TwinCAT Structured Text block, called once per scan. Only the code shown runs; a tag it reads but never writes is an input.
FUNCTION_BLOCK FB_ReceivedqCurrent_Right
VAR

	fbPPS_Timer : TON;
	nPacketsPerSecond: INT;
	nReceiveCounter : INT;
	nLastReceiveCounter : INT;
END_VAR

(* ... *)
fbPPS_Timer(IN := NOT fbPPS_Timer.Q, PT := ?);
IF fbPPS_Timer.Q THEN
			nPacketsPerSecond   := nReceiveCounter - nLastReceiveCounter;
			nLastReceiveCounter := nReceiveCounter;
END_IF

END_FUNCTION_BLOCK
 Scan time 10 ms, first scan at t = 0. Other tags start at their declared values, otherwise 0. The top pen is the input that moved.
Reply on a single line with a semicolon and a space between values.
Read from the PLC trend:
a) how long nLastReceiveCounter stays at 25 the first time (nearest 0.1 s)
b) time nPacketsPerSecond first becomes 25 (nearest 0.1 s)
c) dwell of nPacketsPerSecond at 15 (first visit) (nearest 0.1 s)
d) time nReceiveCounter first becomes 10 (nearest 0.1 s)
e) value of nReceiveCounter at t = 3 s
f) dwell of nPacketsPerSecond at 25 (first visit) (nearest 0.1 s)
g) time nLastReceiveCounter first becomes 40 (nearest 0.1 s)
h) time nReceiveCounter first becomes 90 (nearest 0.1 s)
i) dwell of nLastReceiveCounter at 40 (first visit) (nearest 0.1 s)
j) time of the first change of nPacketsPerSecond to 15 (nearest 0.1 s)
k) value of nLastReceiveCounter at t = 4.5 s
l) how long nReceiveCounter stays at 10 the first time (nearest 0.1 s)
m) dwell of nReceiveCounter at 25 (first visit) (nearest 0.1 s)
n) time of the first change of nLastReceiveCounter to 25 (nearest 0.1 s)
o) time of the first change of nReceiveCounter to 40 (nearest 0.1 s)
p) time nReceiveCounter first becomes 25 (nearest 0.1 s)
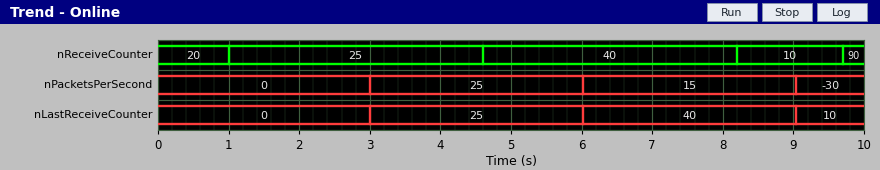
3.0 s; 3.0 s; 3.0 s; 8.2 s; 25; 3.0 s; 6.0 s; 9.7 s; 3.0 s; 6.0 s; 25; 1.5 s; 3.6 s; 3.0 s; 4.6 s; 1.0 s
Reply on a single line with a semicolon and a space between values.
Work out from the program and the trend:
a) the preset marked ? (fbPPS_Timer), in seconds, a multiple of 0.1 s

3.0 s
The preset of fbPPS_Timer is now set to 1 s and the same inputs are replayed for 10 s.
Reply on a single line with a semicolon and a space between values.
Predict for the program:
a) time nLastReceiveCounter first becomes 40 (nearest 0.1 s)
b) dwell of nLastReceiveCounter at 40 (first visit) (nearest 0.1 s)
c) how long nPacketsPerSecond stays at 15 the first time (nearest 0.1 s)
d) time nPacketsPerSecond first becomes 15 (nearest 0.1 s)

5.1 s; 4.1 s; 1.0 s; 5.1 s
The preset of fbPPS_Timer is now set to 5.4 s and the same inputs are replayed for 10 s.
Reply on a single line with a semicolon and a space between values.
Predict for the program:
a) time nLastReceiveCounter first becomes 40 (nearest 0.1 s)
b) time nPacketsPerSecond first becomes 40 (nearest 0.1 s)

5.4 s; 5.4 s
